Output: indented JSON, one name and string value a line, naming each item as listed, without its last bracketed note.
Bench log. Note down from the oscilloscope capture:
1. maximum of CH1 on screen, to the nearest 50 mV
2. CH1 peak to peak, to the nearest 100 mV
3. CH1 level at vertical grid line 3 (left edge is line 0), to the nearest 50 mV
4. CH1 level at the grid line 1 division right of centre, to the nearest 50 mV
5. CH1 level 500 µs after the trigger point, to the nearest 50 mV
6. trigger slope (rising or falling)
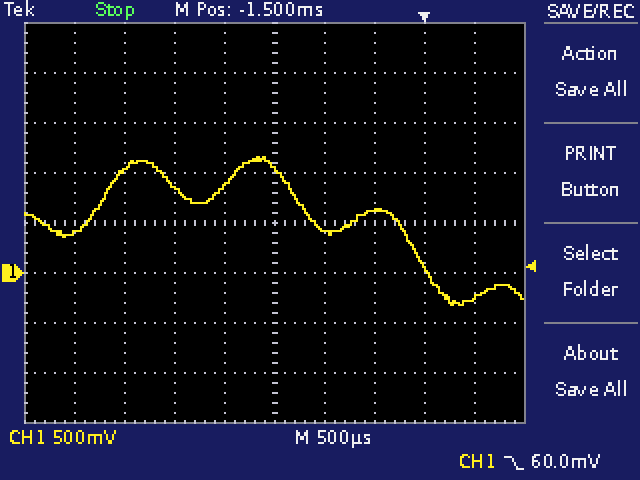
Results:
{
  "maximum of CH1 on screen, to the nearest 50 mV": "1.15 V",
  "CH1 peak to peak, to the nearest 100 mV": "1.50 V",
  "CH1 level at vertical grid line 3 (left edge is line 0), to the nearest 50 mV": "850 mV",
  "CH1 level at the grid line 1 division right of centre, to the nearest 50 mV": "450 mV",
  "CH1 level 500 µs after the trigger point, to the nearest 50 mV": "-250 mV",
  "trigger slope": "falling"
}
